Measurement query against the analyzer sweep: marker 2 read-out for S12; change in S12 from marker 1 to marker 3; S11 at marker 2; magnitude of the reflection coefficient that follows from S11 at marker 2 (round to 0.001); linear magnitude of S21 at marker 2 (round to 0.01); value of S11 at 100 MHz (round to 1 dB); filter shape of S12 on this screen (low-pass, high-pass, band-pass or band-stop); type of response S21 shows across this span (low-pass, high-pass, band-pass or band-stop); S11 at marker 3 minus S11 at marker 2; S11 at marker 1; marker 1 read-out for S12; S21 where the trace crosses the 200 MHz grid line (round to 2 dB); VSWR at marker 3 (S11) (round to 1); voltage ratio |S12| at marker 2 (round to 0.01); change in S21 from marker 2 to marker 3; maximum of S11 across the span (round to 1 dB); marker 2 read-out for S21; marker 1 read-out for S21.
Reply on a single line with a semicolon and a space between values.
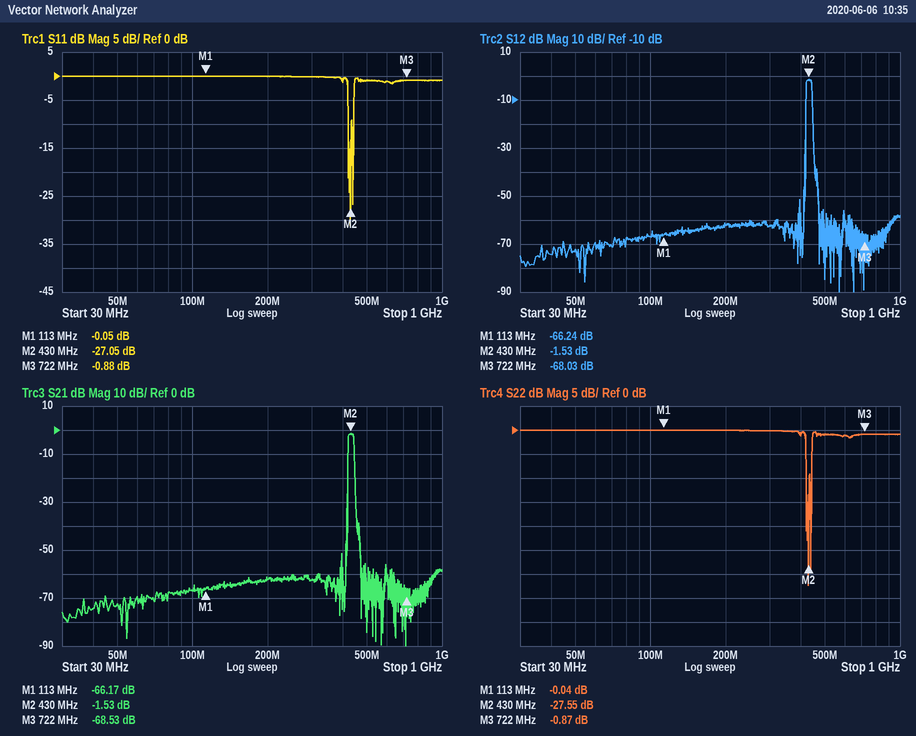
-1.53 dB; -1.79 dB; -27.05 dB; 0.044; 0.84; 0 dB; band-pass; band-pass; 26.17 dB; -0.05 dB; -66.24 dB; -62 dB; 20; 0.84; -67.00 dB; 0 dB; -1.53 dB; -66.17 dB
